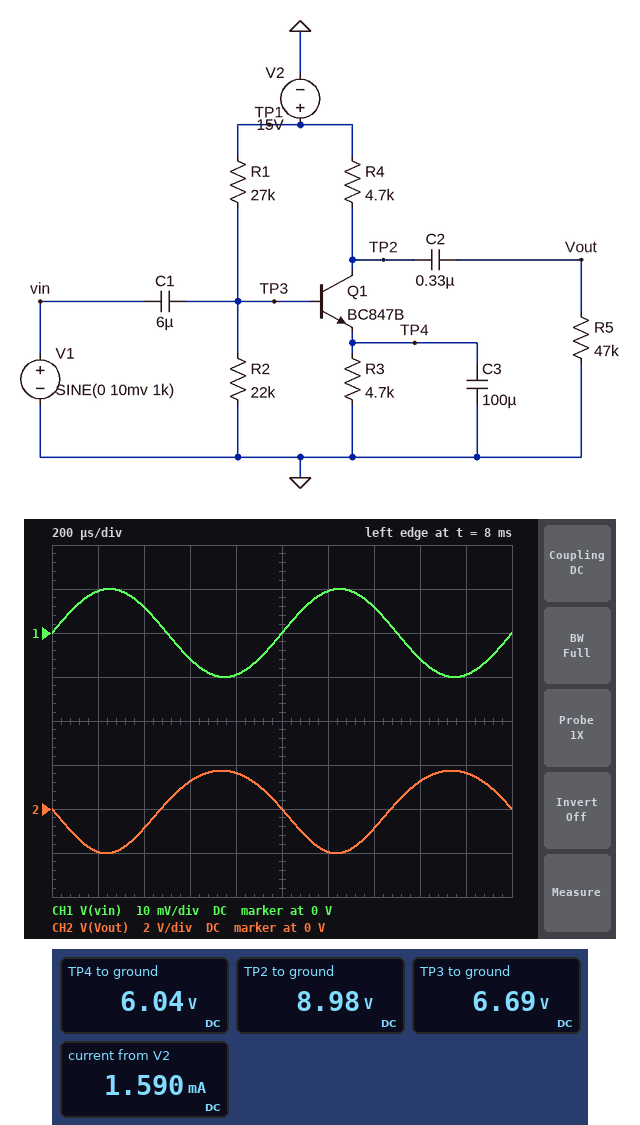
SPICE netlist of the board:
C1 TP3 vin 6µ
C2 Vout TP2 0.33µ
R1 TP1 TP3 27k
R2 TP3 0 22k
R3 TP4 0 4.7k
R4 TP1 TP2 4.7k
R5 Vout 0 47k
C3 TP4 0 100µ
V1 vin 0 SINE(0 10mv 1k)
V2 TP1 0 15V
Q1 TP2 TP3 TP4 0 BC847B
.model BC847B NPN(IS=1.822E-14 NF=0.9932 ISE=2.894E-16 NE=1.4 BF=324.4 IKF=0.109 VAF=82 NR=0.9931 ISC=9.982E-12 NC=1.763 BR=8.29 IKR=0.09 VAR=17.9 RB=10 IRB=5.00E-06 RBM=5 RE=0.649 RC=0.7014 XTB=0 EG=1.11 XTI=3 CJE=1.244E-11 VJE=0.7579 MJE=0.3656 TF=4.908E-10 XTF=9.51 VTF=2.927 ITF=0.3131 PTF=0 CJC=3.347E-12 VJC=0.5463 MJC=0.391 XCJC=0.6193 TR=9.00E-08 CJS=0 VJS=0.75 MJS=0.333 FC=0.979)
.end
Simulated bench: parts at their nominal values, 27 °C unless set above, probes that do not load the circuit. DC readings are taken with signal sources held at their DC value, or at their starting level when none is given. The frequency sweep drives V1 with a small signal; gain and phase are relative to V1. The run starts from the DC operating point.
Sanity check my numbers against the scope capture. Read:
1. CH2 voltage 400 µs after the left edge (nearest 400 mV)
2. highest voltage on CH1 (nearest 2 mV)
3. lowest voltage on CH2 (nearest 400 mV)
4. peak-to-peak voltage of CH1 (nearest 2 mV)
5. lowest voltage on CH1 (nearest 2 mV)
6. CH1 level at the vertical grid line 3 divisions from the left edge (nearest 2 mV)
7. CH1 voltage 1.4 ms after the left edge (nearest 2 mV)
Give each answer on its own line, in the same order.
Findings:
-800 mV
10 mV
-2.0 V
20 mV
-10 mV
-6 mV
6 mV
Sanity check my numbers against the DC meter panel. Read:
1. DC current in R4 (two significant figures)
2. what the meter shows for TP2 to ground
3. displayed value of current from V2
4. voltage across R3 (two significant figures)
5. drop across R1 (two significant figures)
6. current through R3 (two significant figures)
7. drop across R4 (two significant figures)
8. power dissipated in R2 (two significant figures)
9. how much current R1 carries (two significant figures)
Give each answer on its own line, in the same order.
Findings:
1.3 mA
8.98 V
1.590 mA
6.0 V
8.3 V
1.3 mA
6.0 V
2.0 mW
310 µA
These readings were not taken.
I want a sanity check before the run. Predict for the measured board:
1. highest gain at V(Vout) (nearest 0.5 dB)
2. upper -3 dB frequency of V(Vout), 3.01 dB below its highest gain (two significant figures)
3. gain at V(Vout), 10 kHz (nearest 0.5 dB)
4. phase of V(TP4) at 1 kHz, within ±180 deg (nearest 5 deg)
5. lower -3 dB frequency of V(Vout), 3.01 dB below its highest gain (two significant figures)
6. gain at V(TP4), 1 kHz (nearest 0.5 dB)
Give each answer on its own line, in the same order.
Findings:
45.5 dB
18 MHz
45.5 dB
-85 deg
77 Hz
-23.0 dB
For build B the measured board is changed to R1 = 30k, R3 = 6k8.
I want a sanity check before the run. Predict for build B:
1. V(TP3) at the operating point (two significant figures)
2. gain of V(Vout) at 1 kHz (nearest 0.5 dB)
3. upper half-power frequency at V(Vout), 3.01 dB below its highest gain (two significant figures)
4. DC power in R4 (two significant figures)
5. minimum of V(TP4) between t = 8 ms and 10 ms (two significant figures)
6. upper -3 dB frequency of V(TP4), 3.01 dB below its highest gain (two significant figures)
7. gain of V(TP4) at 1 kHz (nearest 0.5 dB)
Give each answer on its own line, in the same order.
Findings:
6.3 V
42.0 dB
24 MHz
3.3 mW
5.7 V
55 Hz
-26.5 dB
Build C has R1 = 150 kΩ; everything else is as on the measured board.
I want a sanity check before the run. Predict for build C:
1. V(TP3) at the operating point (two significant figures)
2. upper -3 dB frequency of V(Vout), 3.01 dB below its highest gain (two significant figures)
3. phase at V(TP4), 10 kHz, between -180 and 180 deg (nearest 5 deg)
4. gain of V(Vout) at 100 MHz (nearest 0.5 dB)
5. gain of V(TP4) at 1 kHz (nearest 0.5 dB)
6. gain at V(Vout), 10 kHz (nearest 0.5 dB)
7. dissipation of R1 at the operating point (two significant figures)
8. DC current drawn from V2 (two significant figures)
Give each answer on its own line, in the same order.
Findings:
1.9 V
36 MHz
-90 deg
23.5 dB
-35.5 dB
33.0 dB
1.1 mW
360 µA
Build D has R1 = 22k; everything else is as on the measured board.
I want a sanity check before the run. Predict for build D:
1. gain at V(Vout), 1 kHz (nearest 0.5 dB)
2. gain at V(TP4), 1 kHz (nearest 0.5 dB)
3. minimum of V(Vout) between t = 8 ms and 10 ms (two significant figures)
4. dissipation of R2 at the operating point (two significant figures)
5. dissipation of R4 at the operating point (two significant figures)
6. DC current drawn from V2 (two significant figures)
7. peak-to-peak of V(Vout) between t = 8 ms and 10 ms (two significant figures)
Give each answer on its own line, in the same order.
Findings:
46.5 dB
-22.0 dB
-1.5 V
2.5 mW
9.8 mW
1.8 mA
3.4 V
